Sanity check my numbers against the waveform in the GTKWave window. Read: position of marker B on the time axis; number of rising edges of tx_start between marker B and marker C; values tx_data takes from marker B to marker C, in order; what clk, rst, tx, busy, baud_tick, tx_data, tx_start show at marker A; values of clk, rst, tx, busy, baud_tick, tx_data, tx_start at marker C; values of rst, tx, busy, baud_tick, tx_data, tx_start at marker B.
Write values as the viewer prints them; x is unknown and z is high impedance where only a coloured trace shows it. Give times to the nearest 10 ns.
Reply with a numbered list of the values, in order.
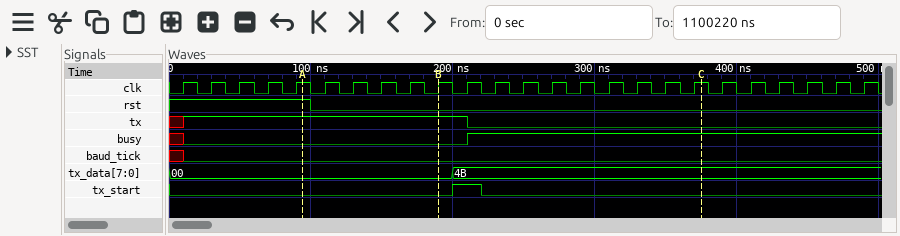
1. 190 ns
2. 1
3. 00, 4B
4. clk=1, rst=1, tx=1, busy=0, baud_tick=0, tx_data=00, tx_start=0
5. clk=1, rst=0, tx=0, busy=1, baud_tick=0, tx_data=4B, tx_start=0
6. rst=0, tx=1, busy=0, baud_tick=0, tx_data=00, tx_start=0
